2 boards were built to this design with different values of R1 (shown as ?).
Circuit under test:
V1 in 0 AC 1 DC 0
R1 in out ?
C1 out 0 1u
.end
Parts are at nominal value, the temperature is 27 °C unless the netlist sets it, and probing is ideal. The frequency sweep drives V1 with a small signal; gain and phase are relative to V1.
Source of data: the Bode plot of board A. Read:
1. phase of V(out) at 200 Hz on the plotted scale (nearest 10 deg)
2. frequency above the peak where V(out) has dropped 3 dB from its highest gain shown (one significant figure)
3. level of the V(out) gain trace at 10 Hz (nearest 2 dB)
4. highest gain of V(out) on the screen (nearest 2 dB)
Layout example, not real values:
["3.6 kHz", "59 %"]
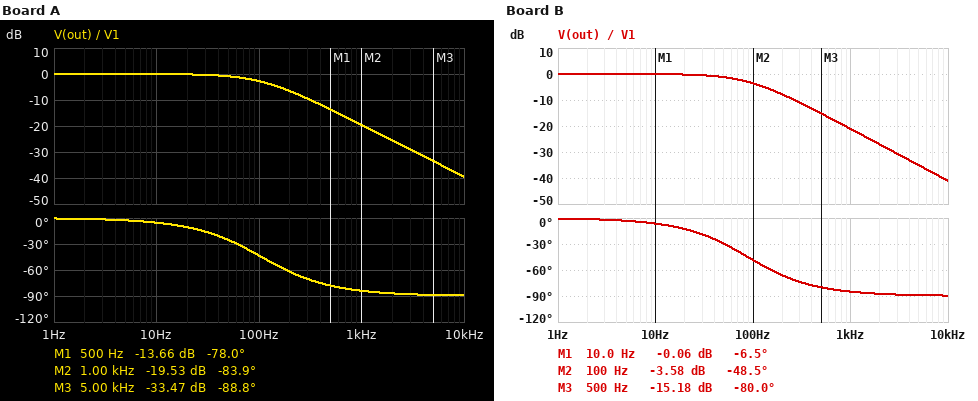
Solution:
["-60 deg", "100 Hz", "0 dB", "0 dB"]
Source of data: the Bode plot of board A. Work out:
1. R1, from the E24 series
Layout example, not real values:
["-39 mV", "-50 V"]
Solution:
["1.5 kΩ"]
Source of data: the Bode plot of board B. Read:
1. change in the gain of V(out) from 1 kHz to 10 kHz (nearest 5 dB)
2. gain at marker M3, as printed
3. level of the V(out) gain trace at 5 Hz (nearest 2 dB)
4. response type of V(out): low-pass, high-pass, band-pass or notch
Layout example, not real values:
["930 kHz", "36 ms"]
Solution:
["-20 dB", "-15.18 dB", "0 dB", "low-pass"]
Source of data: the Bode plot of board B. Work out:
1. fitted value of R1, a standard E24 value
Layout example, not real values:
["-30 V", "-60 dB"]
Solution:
["1.8 kΩ"]
